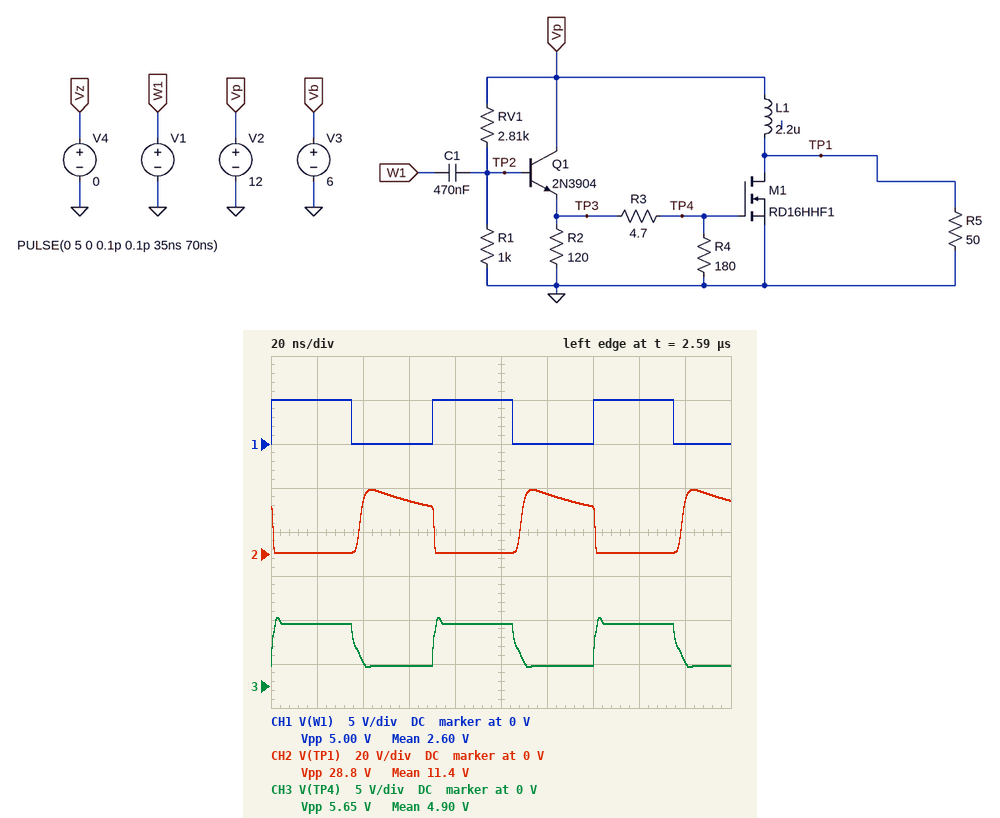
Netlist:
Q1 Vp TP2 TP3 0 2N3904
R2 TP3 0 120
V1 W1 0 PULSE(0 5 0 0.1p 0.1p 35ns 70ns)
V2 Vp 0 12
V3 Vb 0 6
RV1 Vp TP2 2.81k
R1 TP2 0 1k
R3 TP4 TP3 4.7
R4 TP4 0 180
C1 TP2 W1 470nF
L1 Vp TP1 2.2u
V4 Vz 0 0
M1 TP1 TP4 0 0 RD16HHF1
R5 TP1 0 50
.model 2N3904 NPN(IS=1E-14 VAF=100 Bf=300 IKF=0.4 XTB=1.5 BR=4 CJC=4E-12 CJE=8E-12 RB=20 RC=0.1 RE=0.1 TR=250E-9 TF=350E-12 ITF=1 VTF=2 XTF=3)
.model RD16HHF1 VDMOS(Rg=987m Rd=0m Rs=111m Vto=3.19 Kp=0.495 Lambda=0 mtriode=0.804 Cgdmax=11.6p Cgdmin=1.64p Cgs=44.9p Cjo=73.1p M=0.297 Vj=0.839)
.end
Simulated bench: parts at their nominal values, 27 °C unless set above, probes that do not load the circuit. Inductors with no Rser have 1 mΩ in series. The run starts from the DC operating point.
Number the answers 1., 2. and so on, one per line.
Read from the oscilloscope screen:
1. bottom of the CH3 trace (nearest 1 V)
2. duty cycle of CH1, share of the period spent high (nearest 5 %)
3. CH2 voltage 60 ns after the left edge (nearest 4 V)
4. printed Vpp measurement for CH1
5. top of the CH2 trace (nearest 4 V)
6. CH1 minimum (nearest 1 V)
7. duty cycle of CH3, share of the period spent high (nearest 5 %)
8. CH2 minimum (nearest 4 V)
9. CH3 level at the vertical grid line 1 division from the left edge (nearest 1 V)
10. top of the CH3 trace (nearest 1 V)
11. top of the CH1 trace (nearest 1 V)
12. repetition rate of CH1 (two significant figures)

1. 2 V
2. 50 %
3. 24 V
4. 5.00 V
5. 28 V
6. 0 V
7. 50 %
8. 0 V
9. 7 V
10. 8 V
11. 5 V
12. 14 MHz
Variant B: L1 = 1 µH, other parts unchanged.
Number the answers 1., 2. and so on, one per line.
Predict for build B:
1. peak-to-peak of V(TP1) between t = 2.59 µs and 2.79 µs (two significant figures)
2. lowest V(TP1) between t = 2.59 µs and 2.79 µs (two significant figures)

1. 34 V
2. 240 mV
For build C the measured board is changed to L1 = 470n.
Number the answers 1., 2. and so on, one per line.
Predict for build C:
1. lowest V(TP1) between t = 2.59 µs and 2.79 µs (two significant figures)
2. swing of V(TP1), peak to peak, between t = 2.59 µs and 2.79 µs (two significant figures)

1. 200 mV
2. 47 V
